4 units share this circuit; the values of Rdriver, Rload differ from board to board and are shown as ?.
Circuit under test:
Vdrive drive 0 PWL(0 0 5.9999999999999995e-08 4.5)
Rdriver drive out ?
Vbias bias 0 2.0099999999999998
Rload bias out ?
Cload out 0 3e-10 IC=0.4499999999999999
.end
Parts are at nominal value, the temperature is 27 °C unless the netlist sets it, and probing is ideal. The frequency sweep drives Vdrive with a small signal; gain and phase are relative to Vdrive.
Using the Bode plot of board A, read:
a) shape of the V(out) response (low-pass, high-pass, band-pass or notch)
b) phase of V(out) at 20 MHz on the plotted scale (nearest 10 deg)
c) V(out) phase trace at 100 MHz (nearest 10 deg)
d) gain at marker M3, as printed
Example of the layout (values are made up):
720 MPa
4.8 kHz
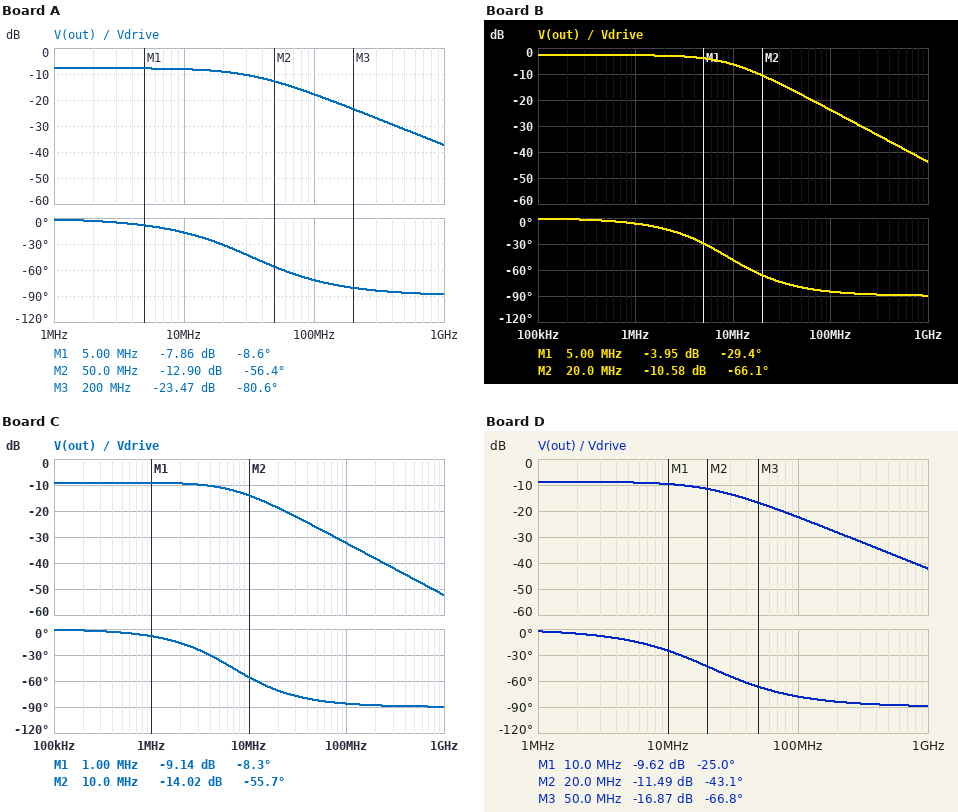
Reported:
low-pass
-30 deg
-70 deg
-23.47 dB
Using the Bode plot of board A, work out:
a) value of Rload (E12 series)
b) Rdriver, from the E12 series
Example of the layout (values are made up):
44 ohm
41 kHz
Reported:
27 Ω
39 Ω
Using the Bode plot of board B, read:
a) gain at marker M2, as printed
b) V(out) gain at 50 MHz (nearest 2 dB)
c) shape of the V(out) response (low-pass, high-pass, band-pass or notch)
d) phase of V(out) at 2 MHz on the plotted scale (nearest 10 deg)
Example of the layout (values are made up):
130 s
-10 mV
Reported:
-10.58 dB
-18 dB
low-pass
-10 deg
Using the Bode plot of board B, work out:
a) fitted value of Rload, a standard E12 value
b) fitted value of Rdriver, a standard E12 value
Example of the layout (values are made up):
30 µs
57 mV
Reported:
220 Ω
82 Ω
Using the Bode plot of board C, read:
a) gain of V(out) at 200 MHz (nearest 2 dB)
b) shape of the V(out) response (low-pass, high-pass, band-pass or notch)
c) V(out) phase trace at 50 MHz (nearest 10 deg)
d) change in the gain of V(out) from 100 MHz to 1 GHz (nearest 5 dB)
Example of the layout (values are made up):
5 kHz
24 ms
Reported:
-38 dB
low-pass
-80 deg
-20 dB
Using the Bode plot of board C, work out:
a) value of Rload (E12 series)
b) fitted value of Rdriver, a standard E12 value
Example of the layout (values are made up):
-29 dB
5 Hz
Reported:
120 Ω
220 Ω
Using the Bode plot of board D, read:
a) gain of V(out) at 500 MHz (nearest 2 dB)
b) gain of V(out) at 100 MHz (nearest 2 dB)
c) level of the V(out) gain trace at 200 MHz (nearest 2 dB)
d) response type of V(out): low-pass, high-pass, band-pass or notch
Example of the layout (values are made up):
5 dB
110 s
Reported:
-36 dB
-22 dB
-28 dB
low-pass
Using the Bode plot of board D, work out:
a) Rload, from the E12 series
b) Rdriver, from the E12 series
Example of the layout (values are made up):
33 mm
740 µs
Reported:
39 Ω
68 Ω
